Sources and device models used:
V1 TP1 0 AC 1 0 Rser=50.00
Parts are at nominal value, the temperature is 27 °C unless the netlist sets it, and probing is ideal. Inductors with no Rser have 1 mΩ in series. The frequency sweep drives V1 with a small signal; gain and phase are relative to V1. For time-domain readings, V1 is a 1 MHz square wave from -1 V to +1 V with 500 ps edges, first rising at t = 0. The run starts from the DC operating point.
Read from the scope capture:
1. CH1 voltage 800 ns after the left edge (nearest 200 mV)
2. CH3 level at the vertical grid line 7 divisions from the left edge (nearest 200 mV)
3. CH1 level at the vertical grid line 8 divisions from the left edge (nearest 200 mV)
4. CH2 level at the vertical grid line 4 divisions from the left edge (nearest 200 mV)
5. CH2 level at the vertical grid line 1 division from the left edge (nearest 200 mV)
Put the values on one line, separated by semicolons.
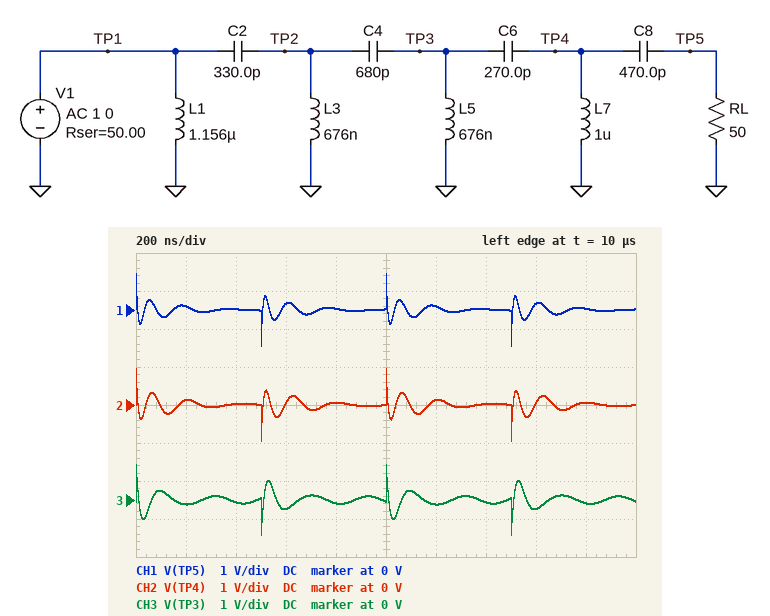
0 V; 0 V; 200 mV; 0 V; 200 mV
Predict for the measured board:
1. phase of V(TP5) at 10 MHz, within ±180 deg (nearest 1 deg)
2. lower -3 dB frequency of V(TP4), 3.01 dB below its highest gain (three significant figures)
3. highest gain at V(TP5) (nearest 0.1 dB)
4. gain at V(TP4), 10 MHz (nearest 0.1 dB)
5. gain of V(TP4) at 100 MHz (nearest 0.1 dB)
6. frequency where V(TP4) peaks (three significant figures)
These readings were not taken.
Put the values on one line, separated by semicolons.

-150 deg; 4.56 MHz; -6.0 dB; -5.4 dB; -6.0 dB; 4.63 MHz
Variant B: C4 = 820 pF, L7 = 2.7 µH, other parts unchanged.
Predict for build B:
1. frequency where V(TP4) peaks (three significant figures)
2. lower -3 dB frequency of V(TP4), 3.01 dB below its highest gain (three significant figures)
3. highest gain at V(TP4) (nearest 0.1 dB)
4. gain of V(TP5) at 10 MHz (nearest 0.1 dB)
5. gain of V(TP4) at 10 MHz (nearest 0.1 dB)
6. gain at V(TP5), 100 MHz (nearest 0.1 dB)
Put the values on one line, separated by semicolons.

4.45 MHz; 4.29 MHz; -1.7 dB; -8.9 dB; -7.3 dB; -6.0 dB
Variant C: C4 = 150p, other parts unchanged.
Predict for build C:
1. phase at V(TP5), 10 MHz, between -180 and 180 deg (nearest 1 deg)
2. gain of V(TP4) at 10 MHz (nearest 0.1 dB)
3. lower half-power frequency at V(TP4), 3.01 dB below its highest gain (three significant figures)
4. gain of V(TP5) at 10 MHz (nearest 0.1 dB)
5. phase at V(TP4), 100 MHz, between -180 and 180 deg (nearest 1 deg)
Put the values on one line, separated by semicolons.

-90 deg; -6.2 dB; 6.94 MHz; -7.8 dB; 21 deg
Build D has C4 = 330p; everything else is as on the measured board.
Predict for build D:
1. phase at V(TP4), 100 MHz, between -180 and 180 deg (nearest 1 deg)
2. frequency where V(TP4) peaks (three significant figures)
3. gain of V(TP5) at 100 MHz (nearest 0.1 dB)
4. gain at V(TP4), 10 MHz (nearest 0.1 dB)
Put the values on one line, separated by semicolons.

18 deg; 6.01 MHz; -6.0 dB; -4.6 dB
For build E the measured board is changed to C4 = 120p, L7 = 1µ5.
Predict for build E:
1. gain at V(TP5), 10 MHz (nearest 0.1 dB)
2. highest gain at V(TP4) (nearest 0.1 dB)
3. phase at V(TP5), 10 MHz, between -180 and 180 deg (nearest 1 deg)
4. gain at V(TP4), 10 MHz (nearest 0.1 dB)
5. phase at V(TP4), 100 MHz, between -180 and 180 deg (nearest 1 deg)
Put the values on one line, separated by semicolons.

-9.3 dB; -5.7 dB; -81 deg; -7.7 dB; 22 deg
